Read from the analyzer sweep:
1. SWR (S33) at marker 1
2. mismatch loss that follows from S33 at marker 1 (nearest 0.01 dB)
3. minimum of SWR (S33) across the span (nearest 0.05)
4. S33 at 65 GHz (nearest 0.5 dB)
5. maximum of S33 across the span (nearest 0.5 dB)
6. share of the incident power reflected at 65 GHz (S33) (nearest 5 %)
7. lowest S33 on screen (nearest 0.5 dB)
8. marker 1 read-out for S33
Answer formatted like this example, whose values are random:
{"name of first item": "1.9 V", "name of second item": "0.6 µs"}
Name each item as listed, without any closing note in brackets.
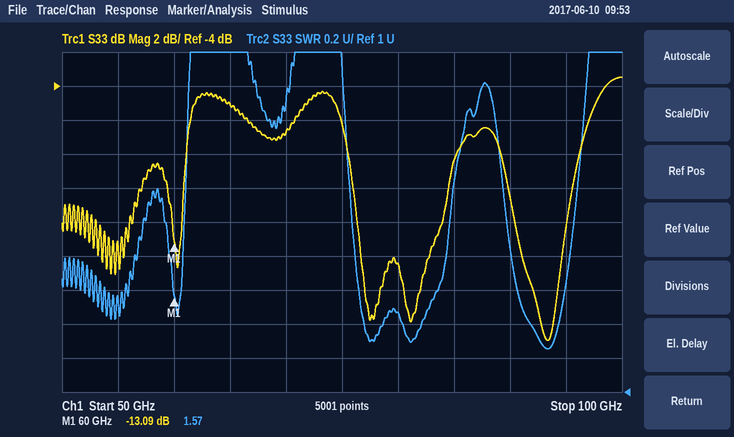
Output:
{"SWR (S33) at marker 1": "1.57", "mismatch loss that follows from S33 at marker 1": "0.22 dB", "minimum of SWR (S33) across the span": "1.25", "S33 at 65 GHz": "-5.0 dB", "maximum of S33 across the span": "-3.5 dB", "share of the incident power reflected at 65 GHz (S33)": "30 %", "lowest S33 on screen": "-19.0 dB", "marker 1 read-out for S33": "-13.09 dB"}
